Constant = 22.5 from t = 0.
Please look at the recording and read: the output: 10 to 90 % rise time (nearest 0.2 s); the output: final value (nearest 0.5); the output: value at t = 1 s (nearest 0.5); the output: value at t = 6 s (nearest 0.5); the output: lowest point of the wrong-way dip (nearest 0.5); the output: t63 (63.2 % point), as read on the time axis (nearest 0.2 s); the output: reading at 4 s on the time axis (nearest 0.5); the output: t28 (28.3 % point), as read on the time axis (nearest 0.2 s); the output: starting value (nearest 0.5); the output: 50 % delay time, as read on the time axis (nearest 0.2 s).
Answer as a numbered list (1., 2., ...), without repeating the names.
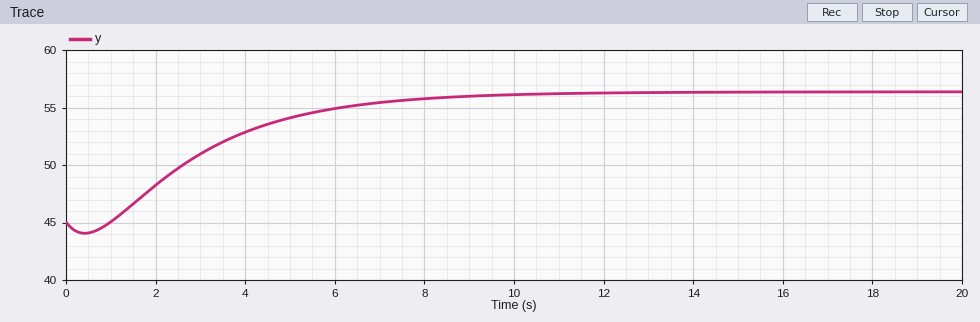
1. 5.2 s
2. 56.5
3. 45.0
4. 55.0
5. 44.0
6. 3.6 s
7. 53.0
8. 2.0 s
9. 45.0
10. 2.8 s
